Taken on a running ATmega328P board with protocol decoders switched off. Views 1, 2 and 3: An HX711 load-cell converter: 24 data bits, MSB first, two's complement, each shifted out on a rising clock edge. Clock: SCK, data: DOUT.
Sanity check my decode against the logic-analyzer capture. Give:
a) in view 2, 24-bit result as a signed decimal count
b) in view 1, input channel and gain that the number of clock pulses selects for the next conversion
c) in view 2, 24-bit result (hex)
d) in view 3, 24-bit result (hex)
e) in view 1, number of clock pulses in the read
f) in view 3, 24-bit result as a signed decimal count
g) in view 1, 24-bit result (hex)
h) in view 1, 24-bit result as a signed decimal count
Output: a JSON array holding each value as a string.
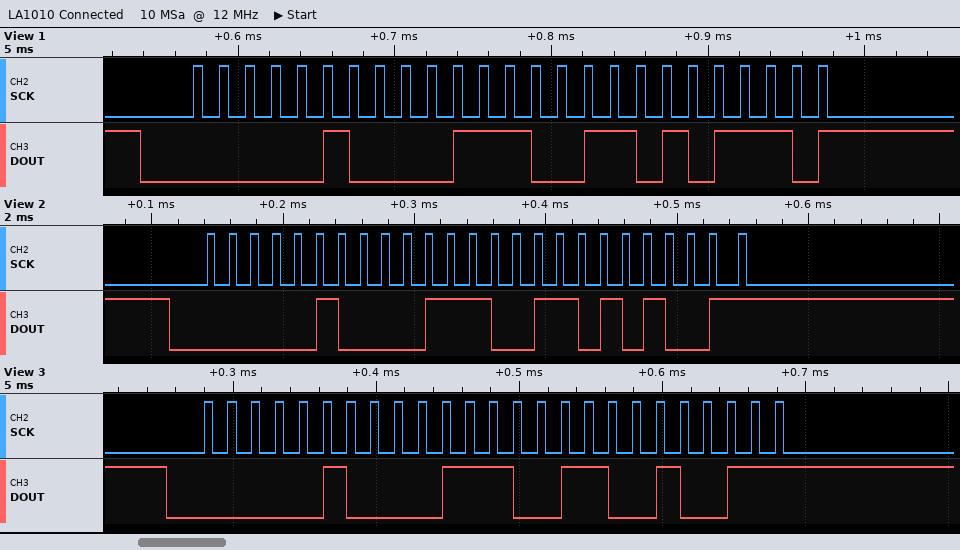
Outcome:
["276905", "channel A, gain 128", "0x0439A9", "0x043993", "25", "276883", "0x0439AE", "276910"]
